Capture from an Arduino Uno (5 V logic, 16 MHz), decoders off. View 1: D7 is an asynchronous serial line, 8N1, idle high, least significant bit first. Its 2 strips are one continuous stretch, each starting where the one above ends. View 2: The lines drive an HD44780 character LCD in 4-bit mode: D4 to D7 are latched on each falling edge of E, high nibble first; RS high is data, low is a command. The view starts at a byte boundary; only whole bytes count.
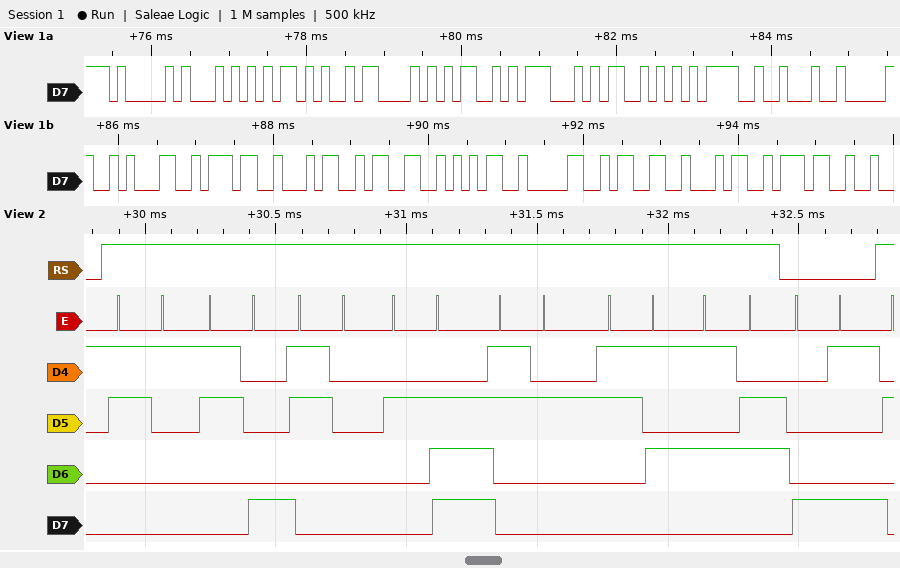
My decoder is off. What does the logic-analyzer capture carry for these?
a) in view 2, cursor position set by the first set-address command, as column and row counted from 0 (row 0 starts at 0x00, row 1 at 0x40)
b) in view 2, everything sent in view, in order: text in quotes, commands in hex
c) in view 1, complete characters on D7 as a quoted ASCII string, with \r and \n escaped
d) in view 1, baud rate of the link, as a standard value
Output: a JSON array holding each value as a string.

["column 9, row 0", "\"180.25V\" 0x89", "\"AT+CMGS=\\\"0174350347\"", "9600 baud"]
